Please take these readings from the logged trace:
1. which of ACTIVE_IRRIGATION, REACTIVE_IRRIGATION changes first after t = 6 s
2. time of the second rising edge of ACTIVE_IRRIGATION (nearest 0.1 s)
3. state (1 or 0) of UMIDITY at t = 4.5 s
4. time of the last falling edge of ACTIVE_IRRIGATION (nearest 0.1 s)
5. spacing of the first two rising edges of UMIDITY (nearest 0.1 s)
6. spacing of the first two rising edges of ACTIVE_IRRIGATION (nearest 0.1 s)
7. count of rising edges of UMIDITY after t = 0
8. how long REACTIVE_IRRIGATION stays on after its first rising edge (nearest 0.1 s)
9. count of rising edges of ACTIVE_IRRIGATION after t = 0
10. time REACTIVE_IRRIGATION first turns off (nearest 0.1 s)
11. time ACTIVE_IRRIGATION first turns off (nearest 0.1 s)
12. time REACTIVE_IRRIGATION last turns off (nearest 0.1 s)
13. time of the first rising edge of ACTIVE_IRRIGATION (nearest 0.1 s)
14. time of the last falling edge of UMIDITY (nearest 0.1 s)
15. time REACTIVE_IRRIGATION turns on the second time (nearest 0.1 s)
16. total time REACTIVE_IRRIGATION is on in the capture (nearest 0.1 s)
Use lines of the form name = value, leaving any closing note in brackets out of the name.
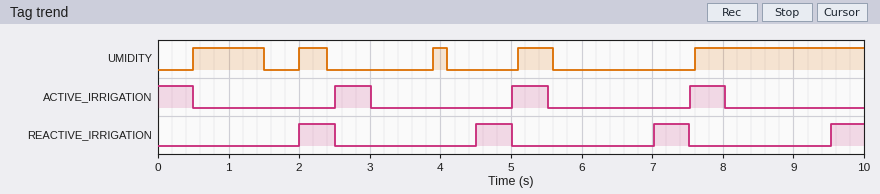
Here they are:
which of ACTIVE_IRRIGATION, REACTIVE_IRRIGATION changes first after t = 6 s = REACTIVE_IRRIGATION
time of the second rising edge of ACTIVE_IRRIGATION = 5.0 s
state (1 or 0) of UMIDITY at t = 4.5 s = 0
time of the last falling edge of ACTIVE_IRRIGATION = 8.0 s
spacing of the first two rising edges of UMIDITY = 1.5 s
spacing of the first two rising edges of ACTIVE_IRRIGATION = 2.5 s
count of rising edges of UMIDITY after t = 0 = 5
how long REACTIVE_IRRIGATION stays on after its first rising edge = 0.5 s
count of rising edges of ACTIVE_IRRIGATION after t = 0 = 3
time REACTIVE_IRRIGATION first turns off = 2.5 s
time ACTIVE_IRRIGATION first turns off = 0.5 s
time REACTIVE_IRRIGATION last turns off = 7.5 s
time of the first rising edge of ACTIVE_IRRIGATION = 2.5 s
time of the last falling edge of UMIDITY = 5.6 s
time REACTIVE_IRRIGATION turns on the second time = 4.5 s
total time REACTIVE_IRRIGATION is on in the capture = 2.0 s
